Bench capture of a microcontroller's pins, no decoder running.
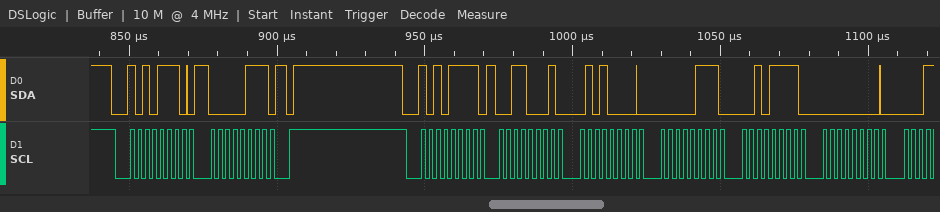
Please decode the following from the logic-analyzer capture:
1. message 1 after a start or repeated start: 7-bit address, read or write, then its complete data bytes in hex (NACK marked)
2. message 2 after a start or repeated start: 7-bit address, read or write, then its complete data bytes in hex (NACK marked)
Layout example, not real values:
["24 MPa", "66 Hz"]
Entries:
["0x57 write: 07", "0x57 read: 31 50 07 2F 00"]
